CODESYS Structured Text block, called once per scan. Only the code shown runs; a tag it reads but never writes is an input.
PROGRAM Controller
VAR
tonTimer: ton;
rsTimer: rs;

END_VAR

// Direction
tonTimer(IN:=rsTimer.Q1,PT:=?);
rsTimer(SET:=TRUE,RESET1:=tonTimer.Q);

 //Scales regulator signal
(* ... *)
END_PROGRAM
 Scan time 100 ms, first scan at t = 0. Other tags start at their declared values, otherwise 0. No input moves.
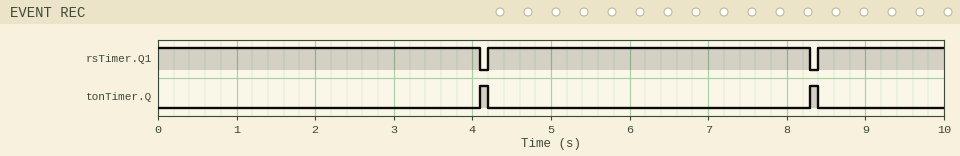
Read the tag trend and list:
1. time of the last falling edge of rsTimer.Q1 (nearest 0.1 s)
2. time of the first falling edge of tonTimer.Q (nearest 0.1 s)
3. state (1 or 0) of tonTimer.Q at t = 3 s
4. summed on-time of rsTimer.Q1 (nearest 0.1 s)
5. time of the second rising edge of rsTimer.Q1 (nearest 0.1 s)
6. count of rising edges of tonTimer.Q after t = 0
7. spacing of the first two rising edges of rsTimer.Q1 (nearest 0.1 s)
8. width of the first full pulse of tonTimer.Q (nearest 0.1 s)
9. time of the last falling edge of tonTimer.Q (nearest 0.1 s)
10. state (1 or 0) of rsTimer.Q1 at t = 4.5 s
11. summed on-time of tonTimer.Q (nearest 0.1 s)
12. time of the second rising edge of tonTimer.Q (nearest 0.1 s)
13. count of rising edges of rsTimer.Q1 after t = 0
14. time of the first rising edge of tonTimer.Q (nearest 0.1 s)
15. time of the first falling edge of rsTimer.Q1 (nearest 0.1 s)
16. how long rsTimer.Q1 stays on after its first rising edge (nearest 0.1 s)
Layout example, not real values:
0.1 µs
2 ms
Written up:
8.3 s
4.2 s
0
9.8 s
8.4 s
2
4.2 s
0.1 s
8.4 s
1
0.2 s
8.3 s
2
4.1 s
4.1 s
4.1 s
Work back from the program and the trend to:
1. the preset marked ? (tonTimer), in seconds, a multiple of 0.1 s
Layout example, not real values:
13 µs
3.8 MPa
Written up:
4.0 s
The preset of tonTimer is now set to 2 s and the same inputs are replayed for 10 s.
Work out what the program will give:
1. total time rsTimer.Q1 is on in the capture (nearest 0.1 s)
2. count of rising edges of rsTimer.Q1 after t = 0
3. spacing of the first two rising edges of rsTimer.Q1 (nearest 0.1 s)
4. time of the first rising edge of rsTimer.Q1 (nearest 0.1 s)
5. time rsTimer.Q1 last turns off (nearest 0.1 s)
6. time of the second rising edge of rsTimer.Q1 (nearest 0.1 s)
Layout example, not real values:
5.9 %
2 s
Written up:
9.6 s
4
2.2 s
2.2 s
8.7 s
4.4 s
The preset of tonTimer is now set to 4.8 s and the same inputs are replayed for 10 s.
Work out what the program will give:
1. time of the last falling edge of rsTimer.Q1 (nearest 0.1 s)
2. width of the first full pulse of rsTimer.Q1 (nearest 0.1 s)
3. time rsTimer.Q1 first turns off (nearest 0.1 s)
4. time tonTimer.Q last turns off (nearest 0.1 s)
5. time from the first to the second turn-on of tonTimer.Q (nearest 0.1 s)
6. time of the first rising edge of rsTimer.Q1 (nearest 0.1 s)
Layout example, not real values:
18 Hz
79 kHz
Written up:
9.9 s
4.9 s
4.9 s
5.0 s
5.0 s
5.0 s
